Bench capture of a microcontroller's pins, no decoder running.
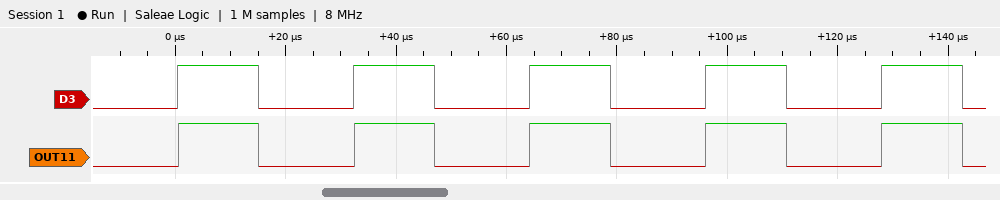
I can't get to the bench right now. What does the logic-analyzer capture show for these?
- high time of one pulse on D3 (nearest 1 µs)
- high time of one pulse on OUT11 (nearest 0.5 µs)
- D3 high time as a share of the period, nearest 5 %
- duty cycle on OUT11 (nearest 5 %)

15 µs
14.5 µs
45 %
45 %
